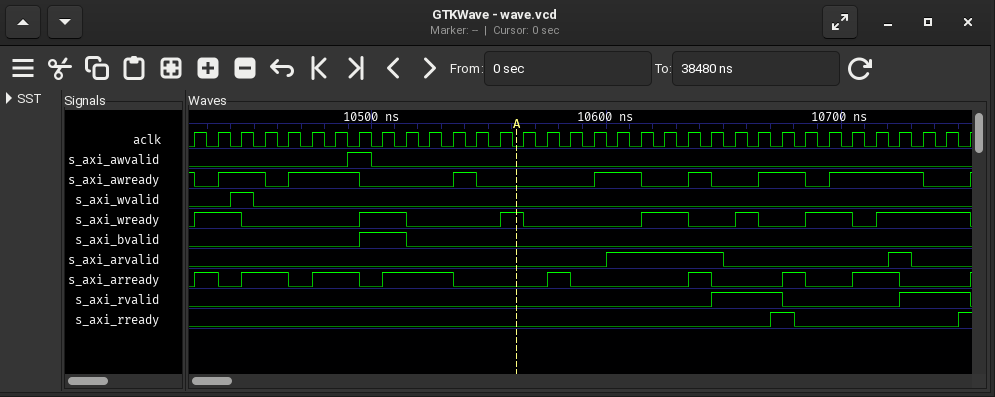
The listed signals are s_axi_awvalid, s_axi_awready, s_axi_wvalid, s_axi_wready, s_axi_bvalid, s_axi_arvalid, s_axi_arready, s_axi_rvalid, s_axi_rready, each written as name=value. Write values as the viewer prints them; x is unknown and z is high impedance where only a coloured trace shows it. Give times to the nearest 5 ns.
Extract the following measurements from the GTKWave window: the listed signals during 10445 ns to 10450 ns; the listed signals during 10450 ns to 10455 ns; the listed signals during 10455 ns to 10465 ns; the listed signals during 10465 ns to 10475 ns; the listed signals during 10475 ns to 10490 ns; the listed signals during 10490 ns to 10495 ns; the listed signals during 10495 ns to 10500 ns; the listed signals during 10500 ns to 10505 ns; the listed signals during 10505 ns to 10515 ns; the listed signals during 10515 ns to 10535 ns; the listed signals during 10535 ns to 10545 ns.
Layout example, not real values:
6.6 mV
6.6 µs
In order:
s_axi_awvalid=0, s_axi_awready=1, s_axi_wvalid=1, s_axi_wready=0, s_axi_bvalid=0, s_axi_arvalid=0, s_axi_arready=1, s_axi_rvalid=0, s_axi_rready=0
s_axi_awvalid=0, s_axi_awready=1, s_axi_wvalid=0, s_axi_wready=0, s_axi_bvalid=0, s_axi_arvalid=0, s_axi_arready=1, s_axi_rvalid=0, s_axi_rready=0
s_axi_awvalid=0, s_axi_awready=0, s_axi_wvalid=0, s_axi_wready=0, s_axi_bvalid=0, s_axi_arvalid=0, s_axi_arready=1, s_axi_rvalid=0, s_axi_rready=0
s_axi_awvalid=0, s_axi_awready=1, s_axi_wvalid=0, s_axi_wready=0, s_axi_bvalid=0, s_axi_arvalid=0, s_axi_arready=0, s_axi_rvalid=0, s_axi_rready=0
s_axi_awvalid=0, s_axi_awready=1, s_axi_wvalid=0, s_axi_wready=0, s_axi_bvalid=0, s_axi_arvalid=0, s_axi_arready=1, s_axi_rvalid=0, s_axi_rready=0
s_axi_awvalid=1, s_axi_awready=1, s_axi_wvalid=0, s_axi_wready=0, s_axi_bvalid=0, s_axi_arvalid=0, s_axi_arready=1, s_axi_rvalid=0, s_axi_rready=0
s_axi_awvalid=1, s_axi_awready=0, s_axi_wvalid=0, s_axi_wready=1, s_axi_bvalid=1, s_axi_arvalid=0, s_axi_arready=0, s_axi_rvalid=0, s_axi_rready=0
s_axi_awvalid=0, s_axi_awready=0, s_axi_wvalid=0, s_axi_wready=1, s_axi_bvalid=1, s_axi_arvalid=0, s_axi_arready=0, s_axi_rvalid=0, s_axi_rready=0
s_axi_awvalid=0, s_axi_awready=0, s_axi_wvalid=0, s_axi_wready=1, s_axi_bvalid=1, s_axi_arvalid=0, s_axi_arready=1, s_axi_rvalid=0, s_axi_rready=0
s_axi_awvalid=0, s_axi_awready=0, s_axi_wvalid=0, s_axi_wready=0, s_axi_bvalid=0, s_axi_arvalid=0, s_axi_arready=1, s_axi_rvalid=0, s_axi_rready=0
s_axi_awvalid=0, s_axi_awready=1, s_axi_wvalid=0, s_axi_wready=0, s_axi_bvalid=0, s_axi_arvalid=0, s_axi_arready=0, s_axi_rvalid=0, s_axi_rready=0
